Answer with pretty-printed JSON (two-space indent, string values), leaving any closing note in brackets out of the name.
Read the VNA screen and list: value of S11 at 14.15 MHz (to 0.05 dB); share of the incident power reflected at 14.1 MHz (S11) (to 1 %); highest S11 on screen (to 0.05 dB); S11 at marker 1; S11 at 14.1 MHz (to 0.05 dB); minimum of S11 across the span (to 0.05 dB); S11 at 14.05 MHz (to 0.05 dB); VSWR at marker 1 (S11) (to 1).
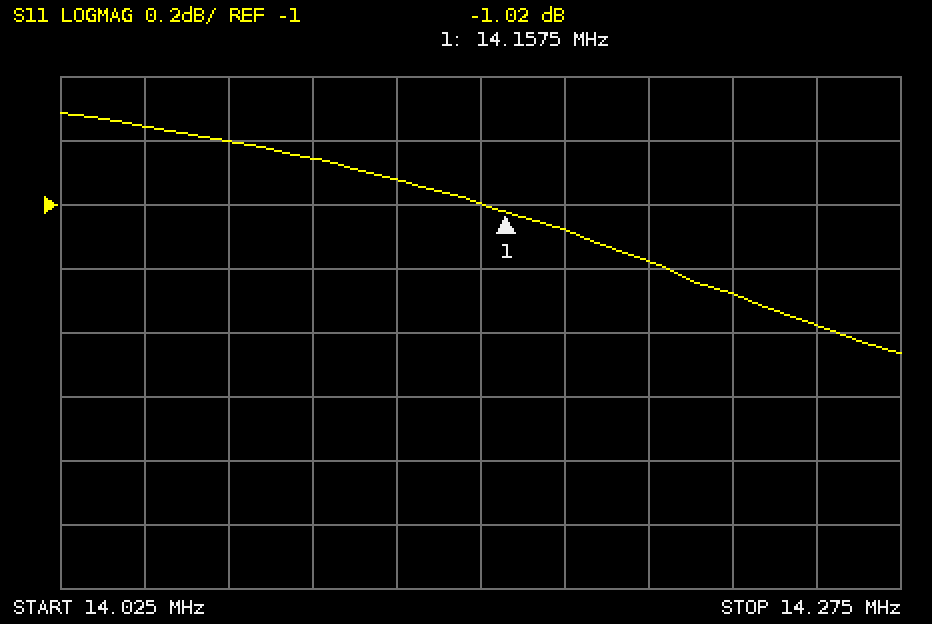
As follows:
{
  "value of S11 at 14.15 MHz": "-1.00 dB",
  "share of the incident power reflected at 14.1 MHz (S11)": "82 %",
  "highest S11 on screen": "-0.70 dB",
  "S11 at marker 1": "-1.02 dB",
  "S11 at 14.1 MHz": "-0.85 dB",
  "minimum of S11 across the span": "-1.45 dB",
  "S11 at 14.05 MHz": "-0.75 dB",
  "VSWR at marker 1 (S11)": "17"
}
